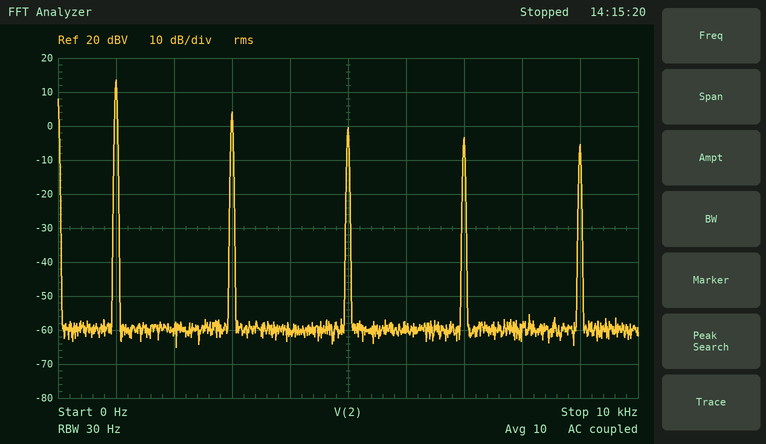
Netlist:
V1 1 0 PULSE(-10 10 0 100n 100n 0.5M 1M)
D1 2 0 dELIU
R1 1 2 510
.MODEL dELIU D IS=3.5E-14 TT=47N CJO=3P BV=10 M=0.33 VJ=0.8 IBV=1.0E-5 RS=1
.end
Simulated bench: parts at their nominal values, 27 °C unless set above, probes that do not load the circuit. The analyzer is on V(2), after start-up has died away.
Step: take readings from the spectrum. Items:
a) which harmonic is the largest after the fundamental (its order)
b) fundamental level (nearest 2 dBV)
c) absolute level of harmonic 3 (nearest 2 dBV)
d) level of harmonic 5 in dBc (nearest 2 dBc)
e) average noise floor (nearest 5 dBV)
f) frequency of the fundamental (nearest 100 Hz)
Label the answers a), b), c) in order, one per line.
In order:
a) 3
b) 14 dBV
c) 4 dBV
d) -14 dBc
e) -60 dBV
f) 1.0 kHz
